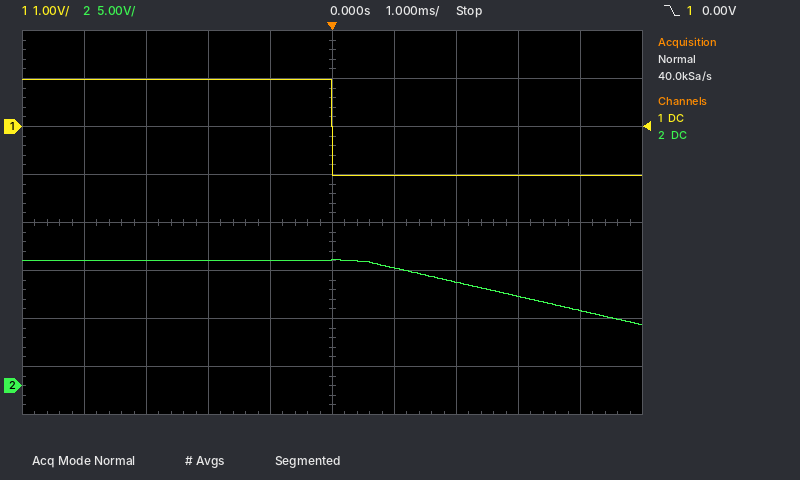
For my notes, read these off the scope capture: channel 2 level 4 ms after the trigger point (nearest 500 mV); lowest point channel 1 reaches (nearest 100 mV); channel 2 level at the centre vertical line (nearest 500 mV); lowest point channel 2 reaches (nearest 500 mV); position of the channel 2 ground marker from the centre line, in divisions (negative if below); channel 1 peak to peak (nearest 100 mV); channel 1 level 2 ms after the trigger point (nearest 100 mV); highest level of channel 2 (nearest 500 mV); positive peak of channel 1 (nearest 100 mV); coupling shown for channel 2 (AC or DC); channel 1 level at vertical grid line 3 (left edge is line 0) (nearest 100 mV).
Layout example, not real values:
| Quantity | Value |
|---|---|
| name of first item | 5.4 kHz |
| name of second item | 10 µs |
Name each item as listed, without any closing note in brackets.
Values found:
| Quantity | Value |
|---|---|
| channel 2 level 4 ms after the trigger point | 8.0 V |
| lowest point channel 1 reaches | -1.0 V |
| channel 2 level at the centre vertical line | 13.0 V |
| lowest point channel 2 reaches | 6.5 V |
| position of the channel 2 ground marker from the centre line, in divisions | -3.4 div |
| channel 1 peak to peak | 2.0 V |
| channel 1 level 2 ms after the trigger point | -1.0 V |
| highest level of channel 2 | 13.0 V |
| positive peak of channel 1 | 1.0 V |
| coupling shown for channel 2 | DC |
| channel 1 level at vertical grid line 3 (left edge is line 0) | 1.0 V |
